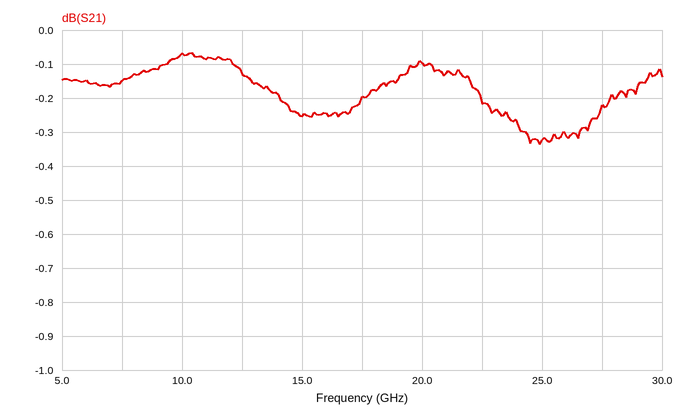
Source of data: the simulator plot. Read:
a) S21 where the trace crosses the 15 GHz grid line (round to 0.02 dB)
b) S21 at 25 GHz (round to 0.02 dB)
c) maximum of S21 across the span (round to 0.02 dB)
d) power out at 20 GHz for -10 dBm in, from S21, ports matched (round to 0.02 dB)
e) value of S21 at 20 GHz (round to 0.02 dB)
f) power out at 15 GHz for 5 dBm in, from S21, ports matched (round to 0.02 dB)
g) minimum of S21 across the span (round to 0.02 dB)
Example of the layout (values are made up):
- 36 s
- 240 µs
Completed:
- -0.26 dB
- -0.32 dB
- -0.06 dB
- -10.10 dBm
- -0.10 dB
- 4.74 dBm
- -0.34 dB
